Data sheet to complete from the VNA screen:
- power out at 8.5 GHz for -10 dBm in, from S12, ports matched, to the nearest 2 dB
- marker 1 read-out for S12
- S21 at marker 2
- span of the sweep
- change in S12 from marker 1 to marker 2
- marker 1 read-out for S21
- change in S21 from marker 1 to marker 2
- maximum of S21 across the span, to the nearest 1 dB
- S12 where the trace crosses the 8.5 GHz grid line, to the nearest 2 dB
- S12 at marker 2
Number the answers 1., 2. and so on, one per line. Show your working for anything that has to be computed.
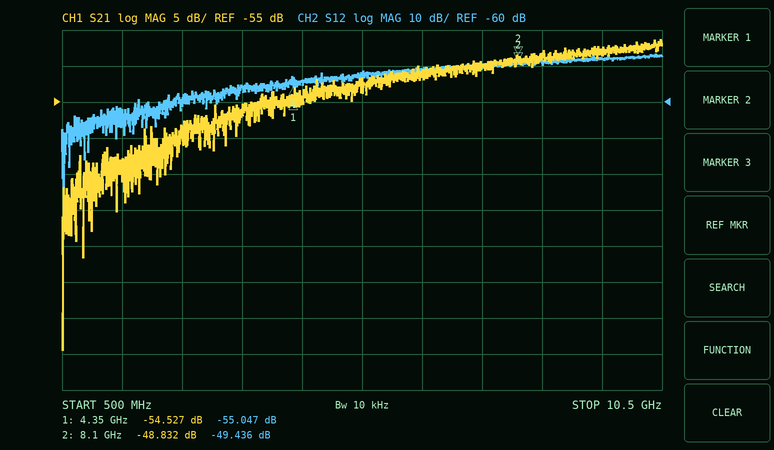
1. -10 dBm + (-50 dB) = -60 dBm
2. -55.047 dB
3. -48.832 dB
4. 10 GHz
5. -49.436 − (-55.047) = 5.611 dB
6. -54.527 dB
7. -48.832 − (-54.527) = 5.695 dB
8. -46 dB
9. -50 dB
10. -49.436 dB
